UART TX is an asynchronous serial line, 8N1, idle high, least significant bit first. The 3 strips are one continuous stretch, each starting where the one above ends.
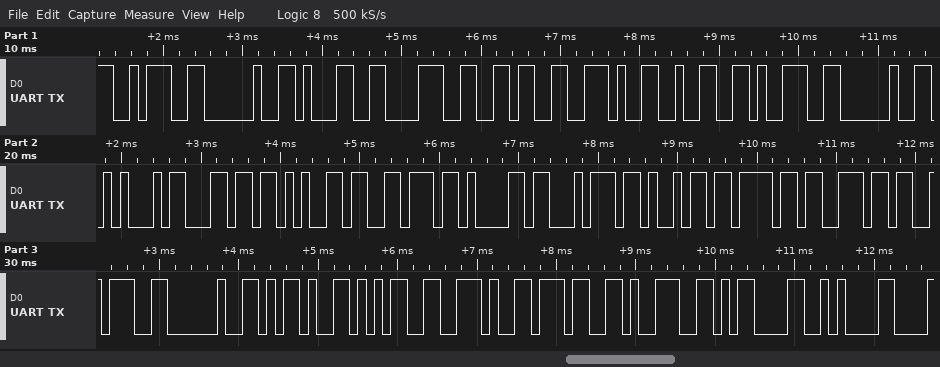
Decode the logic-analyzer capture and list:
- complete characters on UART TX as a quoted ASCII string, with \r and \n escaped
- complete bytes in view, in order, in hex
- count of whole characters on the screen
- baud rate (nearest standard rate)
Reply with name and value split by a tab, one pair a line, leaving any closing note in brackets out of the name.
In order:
complete characters on UART TX as a quoted ASCII string, with \r and \n escaped	": 186.29 Elevation: -5.79\r\n"
complete bytes in view, in order, in hex	3A 20 31 38 36 2E 32 39 20 45 6C 65 76 61 74 69 6F 6E 3A 20 2D 35 2E 37 39 0D 0A
count of whole characters on the screen	27
baud rate	9600 baud
